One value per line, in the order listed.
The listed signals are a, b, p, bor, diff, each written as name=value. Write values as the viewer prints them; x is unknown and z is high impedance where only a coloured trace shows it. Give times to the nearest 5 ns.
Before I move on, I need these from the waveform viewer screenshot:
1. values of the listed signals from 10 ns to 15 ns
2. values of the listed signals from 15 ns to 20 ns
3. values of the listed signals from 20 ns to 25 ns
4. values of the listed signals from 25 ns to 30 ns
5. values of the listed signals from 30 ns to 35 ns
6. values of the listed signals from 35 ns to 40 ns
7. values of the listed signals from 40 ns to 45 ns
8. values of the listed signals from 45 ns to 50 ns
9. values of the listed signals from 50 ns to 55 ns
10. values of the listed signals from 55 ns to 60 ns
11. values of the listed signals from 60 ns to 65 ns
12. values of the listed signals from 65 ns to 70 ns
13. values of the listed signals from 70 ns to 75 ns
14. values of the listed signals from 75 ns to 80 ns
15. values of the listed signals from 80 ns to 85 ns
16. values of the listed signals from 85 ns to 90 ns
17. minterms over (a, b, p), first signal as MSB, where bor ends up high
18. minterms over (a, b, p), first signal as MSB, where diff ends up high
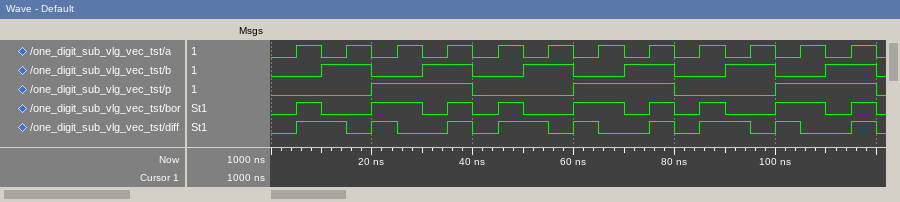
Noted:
a=0, b=1, p=0, bor=0, diff=1
a=1, b=1, p=0, bor=0, diff=0
a=0, b=0, p=1, bor=1, diff=1
a=1, b=0, p=1, bor=1, diff=0
a=0, b=1, p=1, bor=0, diff=0
a=1, b=1, p=1, bor=1, diff=1
a=0, b=0, p=0, bor=0, diff=0
a=1, b=0, p=0, bor=1, diff=1
a=0, b=1, p=0, bor=0, diff=1
a=1, b=1, p=0, bor=0, diff=0
a=0, b=0, p=1, bor=1, diff=1
a=1, b=0, p=1, bor=1, diff=0
a=0, b=1, p=1, bor=0, diff=0
a=1, b=1, p=1, bor=1, diff=1
a=0, b=0, p=0, bor=0, diff=0
a=1, b=0, p=0, bor=1, diff=1
1, 4, 5, 7
1, 2, 4, 7
